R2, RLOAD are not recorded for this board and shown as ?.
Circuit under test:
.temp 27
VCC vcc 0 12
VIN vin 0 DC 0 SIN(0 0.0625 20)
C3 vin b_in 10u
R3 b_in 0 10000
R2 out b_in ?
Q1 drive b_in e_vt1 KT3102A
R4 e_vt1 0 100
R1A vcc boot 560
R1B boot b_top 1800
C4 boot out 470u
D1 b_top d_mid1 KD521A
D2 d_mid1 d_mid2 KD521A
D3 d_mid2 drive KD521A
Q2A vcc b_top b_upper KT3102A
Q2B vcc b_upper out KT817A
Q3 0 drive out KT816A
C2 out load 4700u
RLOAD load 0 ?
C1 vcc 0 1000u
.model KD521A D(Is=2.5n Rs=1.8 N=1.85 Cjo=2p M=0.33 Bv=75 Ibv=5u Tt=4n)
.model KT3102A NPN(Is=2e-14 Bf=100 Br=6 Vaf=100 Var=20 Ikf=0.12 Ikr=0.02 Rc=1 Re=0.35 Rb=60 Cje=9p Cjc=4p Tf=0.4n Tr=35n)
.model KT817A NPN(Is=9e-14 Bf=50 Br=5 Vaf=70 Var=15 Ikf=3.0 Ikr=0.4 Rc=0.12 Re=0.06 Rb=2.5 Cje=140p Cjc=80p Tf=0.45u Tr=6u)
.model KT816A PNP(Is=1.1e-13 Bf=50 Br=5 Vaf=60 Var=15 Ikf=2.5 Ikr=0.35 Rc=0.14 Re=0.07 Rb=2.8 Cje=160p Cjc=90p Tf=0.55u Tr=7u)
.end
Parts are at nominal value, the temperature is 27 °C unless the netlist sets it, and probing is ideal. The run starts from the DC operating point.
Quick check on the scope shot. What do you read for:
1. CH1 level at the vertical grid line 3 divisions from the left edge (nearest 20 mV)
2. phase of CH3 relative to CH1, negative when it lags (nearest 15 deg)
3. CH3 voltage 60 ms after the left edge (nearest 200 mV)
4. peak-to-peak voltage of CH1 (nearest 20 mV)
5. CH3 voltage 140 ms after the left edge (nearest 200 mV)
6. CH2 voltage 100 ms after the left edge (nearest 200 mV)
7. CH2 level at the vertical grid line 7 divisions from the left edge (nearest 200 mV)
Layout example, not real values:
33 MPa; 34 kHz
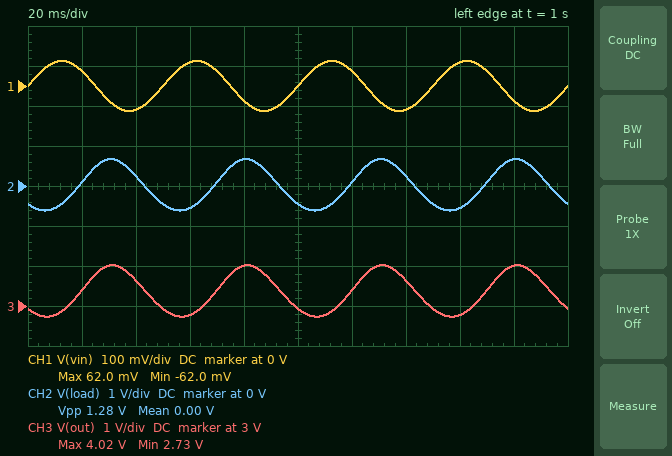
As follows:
60 mV; -135 deg; 2.8 V; 120 mV; 3.6 V; -400 mV; 200 mV
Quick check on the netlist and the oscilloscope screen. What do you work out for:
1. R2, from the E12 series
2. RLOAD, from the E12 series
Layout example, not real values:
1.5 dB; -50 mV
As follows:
15 kΩ; 22 Ω
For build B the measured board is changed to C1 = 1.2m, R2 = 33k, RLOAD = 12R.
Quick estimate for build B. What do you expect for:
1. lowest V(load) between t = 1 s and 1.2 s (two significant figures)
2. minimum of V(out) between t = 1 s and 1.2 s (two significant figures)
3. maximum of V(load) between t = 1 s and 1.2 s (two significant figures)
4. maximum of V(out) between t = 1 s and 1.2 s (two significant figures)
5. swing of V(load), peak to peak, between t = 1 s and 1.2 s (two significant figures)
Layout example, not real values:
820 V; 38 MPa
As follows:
-460 mV; 4.7 V; 620 mV; 5.8 V; 1.1 V
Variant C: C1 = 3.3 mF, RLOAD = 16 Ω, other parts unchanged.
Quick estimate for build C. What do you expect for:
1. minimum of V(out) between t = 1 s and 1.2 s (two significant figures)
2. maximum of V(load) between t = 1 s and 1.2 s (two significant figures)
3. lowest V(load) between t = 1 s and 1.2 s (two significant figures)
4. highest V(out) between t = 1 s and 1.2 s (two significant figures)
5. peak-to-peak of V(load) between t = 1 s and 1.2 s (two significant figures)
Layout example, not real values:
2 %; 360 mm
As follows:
2.8 V; 560 mV; -500 mV; 3.9 V; 1.1 V
